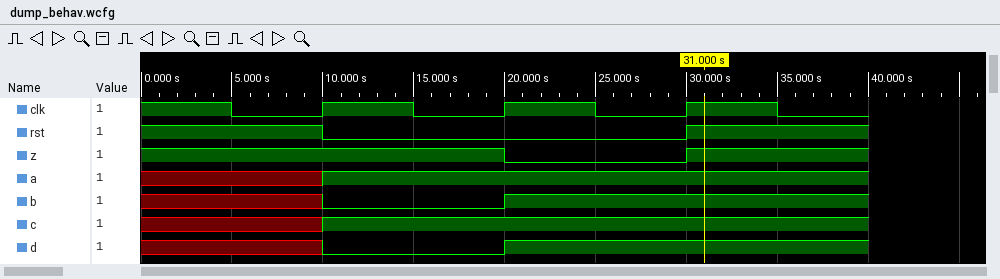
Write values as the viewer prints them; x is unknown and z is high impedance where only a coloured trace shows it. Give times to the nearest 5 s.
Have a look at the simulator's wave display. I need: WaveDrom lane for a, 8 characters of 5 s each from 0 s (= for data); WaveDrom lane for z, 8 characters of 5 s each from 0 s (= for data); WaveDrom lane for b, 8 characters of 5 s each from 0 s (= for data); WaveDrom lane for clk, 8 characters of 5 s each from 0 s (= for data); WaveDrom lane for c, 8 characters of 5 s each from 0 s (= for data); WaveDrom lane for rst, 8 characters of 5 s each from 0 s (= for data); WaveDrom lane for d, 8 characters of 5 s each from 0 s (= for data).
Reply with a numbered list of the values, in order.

1. {name: 'a', wave: 'x.1.....'}
2. {name: 'z', wave: '1...0.1.'}
3. {name: 'b', wave: 'x.0.1...'}
4. {name: 'clk', wave: '10101010'}
5. {name: 'c', wave: 'x.1.....'}
6. {name: 'rst', wave: '1.0...1.'}
7. {name: 'd', wave: 'x.0.1...'}
